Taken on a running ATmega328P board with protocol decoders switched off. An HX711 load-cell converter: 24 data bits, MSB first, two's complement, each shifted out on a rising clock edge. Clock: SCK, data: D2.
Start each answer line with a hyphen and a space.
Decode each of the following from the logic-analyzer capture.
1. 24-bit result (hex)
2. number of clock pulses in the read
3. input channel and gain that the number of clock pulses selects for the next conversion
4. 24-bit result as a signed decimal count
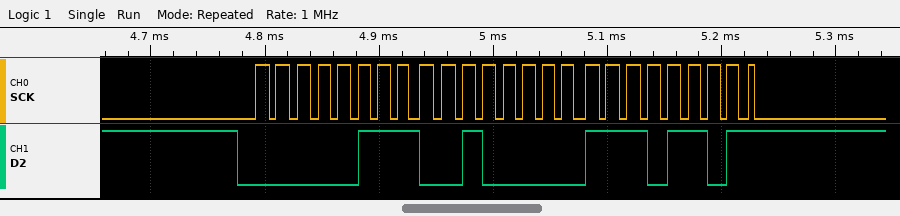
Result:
- 0x0720ED
- 25
- channel A, gain 128
- 467181
